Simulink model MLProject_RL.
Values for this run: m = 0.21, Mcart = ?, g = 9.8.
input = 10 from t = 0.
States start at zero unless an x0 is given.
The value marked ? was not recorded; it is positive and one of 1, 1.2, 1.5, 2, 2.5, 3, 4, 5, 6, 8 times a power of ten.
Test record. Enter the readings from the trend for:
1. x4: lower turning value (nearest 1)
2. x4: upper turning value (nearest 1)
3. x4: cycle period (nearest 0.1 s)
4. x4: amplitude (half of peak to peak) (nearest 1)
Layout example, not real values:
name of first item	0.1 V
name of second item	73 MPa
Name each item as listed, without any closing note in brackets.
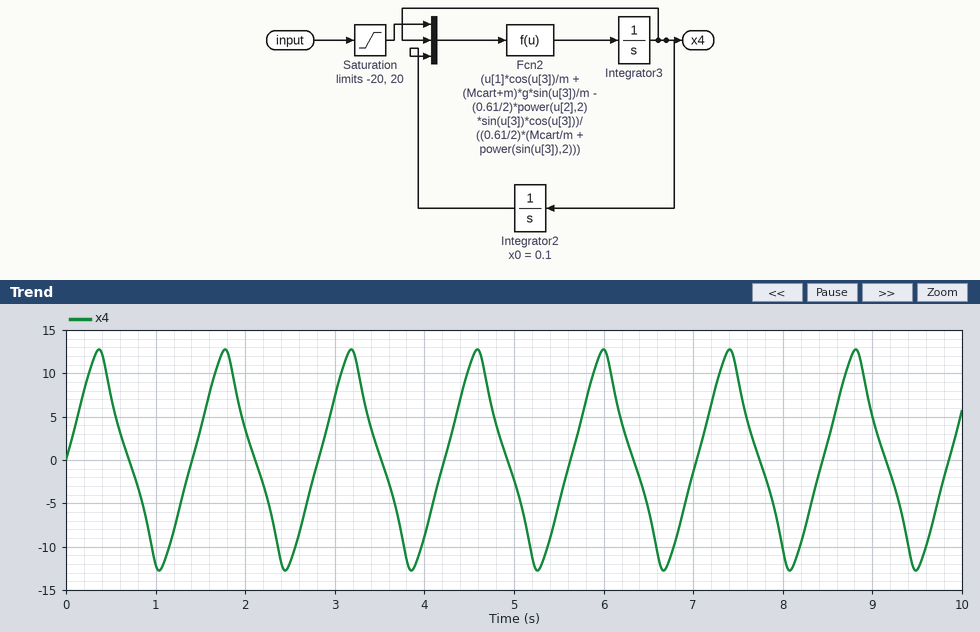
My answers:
x4: lower turning value	-13
x4: upper turning value	13
x4: cycle period	1.4 s
x4: amplitude (half of peak to peak)	13
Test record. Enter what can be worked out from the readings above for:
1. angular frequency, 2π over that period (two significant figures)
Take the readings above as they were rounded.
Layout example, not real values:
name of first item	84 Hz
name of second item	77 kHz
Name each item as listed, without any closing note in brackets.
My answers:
angular frequency, 2π over that period	4.5 rad/s
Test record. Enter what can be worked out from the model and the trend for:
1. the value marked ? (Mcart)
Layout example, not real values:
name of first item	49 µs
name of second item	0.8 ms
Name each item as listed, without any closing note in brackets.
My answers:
the value marked ?	1
